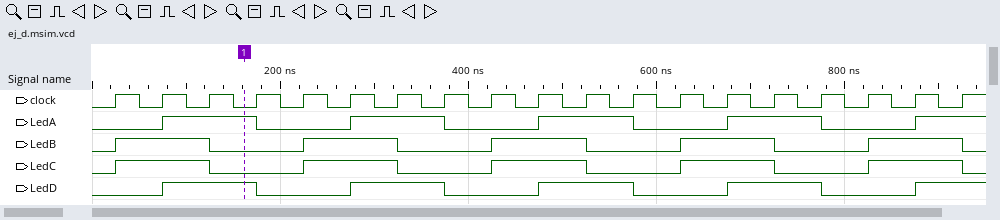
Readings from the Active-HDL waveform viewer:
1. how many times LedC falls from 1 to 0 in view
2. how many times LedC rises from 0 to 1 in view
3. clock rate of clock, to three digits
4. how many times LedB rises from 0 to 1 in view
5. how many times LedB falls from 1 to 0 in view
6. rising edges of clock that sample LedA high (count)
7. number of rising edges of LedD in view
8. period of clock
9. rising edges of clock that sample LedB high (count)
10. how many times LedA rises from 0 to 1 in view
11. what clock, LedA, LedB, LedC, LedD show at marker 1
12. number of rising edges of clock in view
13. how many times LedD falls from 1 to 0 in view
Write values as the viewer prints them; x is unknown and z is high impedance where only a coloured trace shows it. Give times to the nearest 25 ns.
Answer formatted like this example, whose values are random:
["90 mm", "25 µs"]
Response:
["5", "5", "20.0 MHz", "5", "5", "9", "5", "50 ns", "10", "5", "clock=0, LedA=1, LedB=0, LedC=0, LedD=1", "19", "4"]
